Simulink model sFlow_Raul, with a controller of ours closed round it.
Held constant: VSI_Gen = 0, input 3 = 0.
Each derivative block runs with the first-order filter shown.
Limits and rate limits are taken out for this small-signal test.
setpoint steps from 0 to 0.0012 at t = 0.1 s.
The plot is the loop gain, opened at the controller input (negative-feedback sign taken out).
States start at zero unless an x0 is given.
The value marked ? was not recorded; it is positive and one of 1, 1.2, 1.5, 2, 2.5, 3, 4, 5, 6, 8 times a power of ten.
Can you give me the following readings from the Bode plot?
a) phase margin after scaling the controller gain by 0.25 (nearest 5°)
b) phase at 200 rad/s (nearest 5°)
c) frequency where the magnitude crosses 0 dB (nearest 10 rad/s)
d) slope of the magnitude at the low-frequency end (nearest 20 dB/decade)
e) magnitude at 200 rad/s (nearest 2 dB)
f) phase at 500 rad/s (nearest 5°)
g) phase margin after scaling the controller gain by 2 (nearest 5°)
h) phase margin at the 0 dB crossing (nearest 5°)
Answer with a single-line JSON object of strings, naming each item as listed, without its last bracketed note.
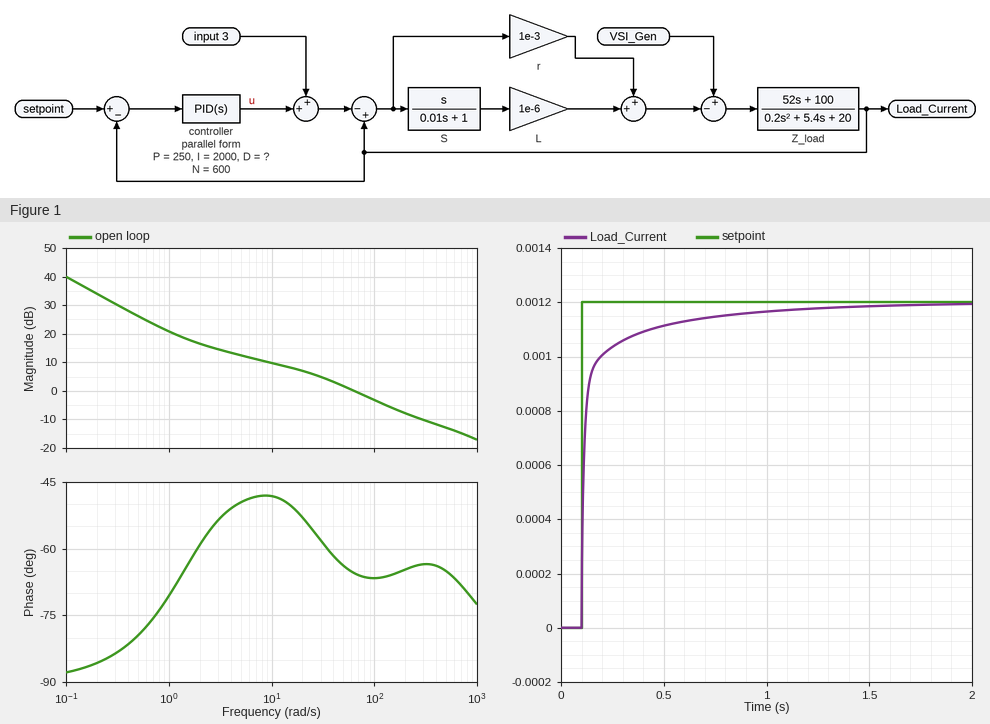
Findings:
{"phase margin after scaling the controller gain by 0.25": "130°", "phase at 200 rad/s": "-65°", "frequency where the magnitude crosses 0 dB": "60 rad/s", "slope of the magnitude at the low-frequency end": "-20 dB/decade", "magnitude at 200 rad/s": "-8 dB", "phase at 500 rad/s": "-65°", "phase margin after scaling the controller gain by 2": "115°", "phase margin at the 0 dB crossing": "115°"}
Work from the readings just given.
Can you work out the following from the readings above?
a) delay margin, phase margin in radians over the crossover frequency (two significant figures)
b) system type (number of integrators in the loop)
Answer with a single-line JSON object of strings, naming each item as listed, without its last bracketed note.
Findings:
{"delay margin, phase margin in radians over the crossover frequency": "0.033 s", "system type": "1"}
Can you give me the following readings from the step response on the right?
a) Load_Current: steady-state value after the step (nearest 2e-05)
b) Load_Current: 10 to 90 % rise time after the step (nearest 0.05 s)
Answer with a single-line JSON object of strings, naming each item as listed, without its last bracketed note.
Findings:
{"Load_Current: steady-state value after the step": "0.00120", "Load_Current: 10 to 90 % rise time after the step": "0.25 s"}
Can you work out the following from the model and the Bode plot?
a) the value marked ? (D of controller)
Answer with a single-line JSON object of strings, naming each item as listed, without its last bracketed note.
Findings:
{"the value marked ?": "0.5"}
